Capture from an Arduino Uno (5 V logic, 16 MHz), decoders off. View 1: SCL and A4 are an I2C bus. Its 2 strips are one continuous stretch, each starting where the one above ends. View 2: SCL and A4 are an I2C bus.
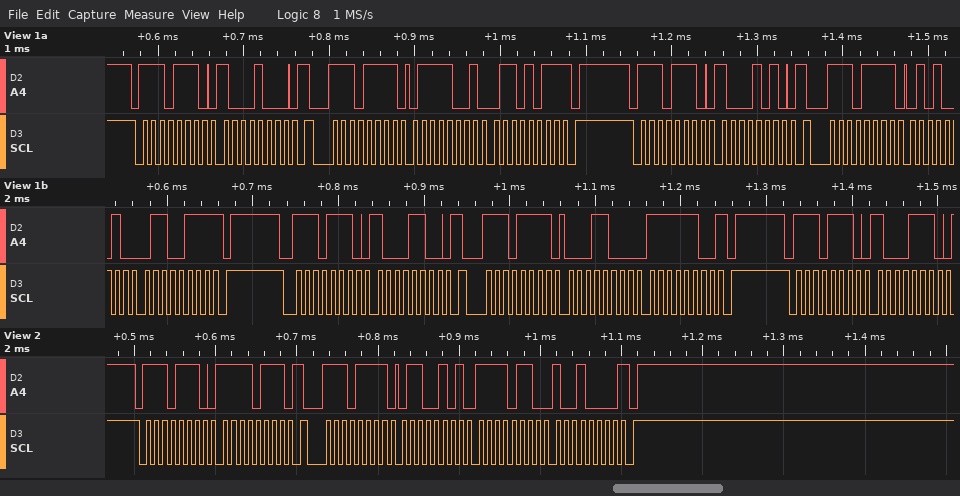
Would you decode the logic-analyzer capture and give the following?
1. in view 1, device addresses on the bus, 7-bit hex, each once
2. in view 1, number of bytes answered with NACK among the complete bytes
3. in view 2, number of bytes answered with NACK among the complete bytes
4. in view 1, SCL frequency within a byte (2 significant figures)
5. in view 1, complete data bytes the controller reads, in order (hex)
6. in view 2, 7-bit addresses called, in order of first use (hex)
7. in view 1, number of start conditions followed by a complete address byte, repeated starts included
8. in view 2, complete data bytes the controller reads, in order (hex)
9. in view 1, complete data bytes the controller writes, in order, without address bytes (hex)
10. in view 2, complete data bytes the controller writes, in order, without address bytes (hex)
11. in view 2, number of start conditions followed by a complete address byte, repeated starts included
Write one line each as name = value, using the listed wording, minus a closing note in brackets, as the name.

in view 1, device addresses on the bus, 7-bit hex, each once = 0x77
in view 1, number of bytes answered with NACK among the complete bytes = 3
in view 2, number of bytes answered with NACK among the complete bytes = 1
in view 1, SCL frequency within a byte = 100 kHz
in view 1, complete data bytes the controller reads, in order = 79 6B 52 67 18 FC
in view 2, 7-bit addresses called, in order of first use = 0x77
in view 1, number of start conditions followed by a complete address byte, repeated starts included = 7
in view 2, complete data bytes the controller reads, in order = 65 F6 90
in view 1, complete data bytes the controller writes, in order, without address bytes = 88 8A 8C 8E
in view 2, complete data bytes the controller writes, in order, without address bytes = F7
in view 2, number of start conditions followed by a complete address byte, repeated starts included = 2
